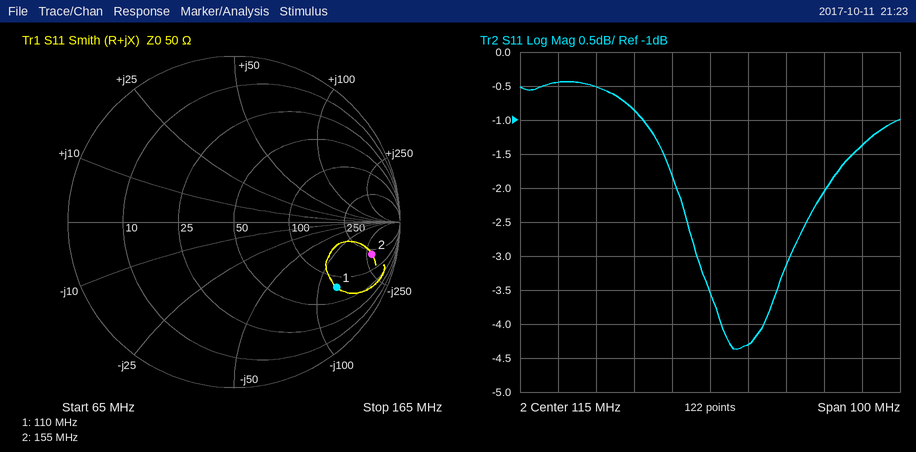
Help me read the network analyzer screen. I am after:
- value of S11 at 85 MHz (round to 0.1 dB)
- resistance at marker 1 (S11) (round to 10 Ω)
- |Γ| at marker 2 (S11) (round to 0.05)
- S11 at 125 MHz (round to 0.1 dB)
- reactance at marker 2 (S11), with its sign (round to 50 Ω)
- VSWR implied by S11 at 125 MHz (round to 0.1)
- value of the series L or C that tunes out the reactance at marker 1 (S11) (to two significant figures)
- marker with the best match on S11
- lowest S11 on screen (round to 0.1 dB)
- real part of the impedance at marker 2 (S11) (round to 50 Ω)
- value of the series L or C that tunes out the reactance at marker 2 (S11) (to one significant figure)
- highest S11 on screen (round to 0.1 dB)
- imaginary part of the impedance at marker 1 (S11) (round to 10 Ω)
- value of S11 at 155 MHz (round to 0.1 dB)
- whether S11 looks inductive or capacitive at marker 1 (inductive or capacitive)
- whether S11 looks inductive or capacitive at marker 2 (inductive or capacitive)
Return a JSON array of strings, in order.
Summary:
["-0.5 dB", "80 Ω", "0.85", "-4.3 dB", "-300 Ω", "4.1", "190 nH", "marker 1", "-4.4 dB", "200 Ω", "300 nH", "-0.4 dB", "-130 Ω", "-1.4 dB", "capacitive", "capacitive"]
